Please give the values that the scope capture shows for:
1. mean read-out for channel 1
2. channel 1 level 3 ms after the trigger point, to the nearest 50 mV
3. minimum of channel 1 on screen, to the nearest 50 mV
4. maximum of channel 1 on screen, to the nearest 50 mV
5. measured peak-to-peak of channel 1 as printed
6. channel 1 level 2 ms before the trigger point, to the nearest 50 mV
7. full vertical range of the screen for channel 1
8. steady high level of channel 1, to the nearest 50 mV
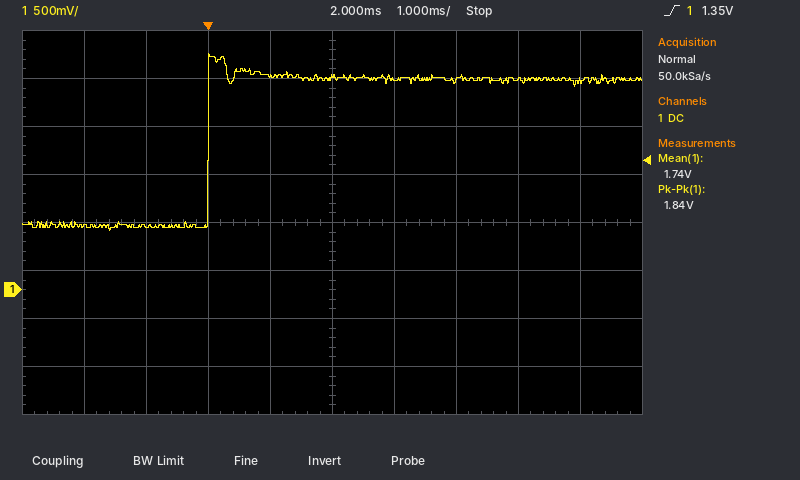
1.74 V
2.20 V
600 mV
2.45 V
1.84 V
650 mV
4 V
2.20 V
